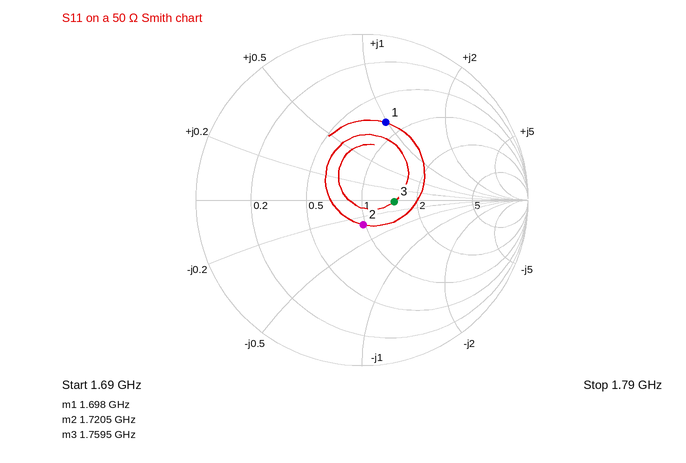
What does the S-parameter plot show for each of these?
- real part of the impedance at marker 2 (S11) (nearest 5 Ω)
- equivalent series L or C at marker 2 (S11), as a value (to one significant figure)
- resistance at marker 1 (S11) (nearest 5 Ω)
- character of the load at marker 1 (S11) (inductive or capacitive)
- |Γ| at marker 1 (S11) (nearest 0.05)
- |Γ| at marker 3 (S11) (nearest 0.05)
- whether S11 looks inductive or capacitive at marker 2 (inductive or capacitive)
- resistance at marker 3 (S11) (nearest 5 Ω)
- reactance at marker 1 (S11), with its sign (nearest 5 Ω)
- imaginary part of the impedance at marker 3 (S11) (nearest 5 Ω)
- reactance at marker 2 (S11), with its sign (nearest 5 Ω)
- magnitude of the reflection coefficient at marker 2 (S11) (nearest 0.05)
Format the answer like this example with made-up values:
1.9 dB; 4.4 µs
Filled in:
50 Ω; 6 pF; 40 Ω; inductive; 0.50; 0.20; capacitive; 75 Ω; +50 Ω; 0 Ω; -15 Ω; 0.15
